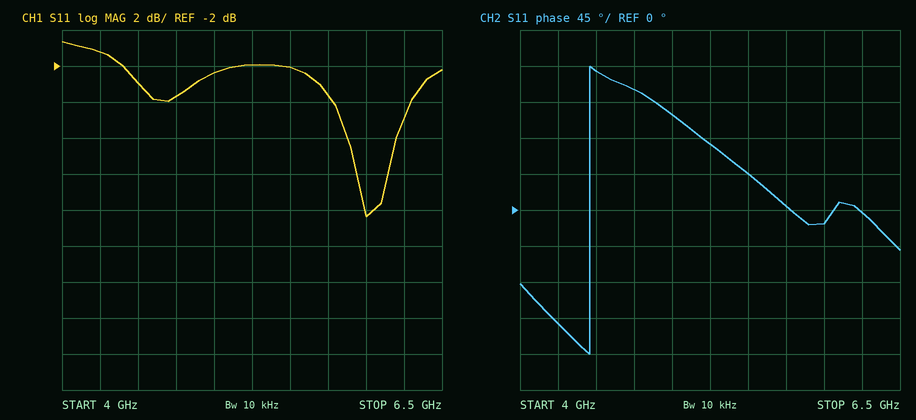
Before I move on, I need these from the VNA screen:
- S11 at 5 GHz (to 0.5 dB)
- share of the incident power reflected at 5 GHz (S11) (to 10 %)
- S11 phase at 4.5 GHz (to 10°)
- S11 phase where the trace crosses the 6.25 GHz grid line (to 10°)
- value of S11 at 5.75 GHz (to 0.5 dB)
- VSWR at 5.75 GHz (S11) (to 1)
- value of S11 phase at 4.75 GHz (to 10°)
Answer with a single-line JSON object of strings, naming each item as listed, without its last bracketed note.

{"S11 at 5 GHz": "-2.5 dB", "share of the incident power reflected at 5 GHz (S11)": "60 %", "S11 phase at 4.5 GHz": "170°", "S11 phase where the trace crosses the 6.25 GHz grid line": "0°", "value of S11 at 5.75 GHz": "-3.5 dB", "VSWR at 5.75 GHz (S11)": "5", "value of S11 phase at 4.75 GHz": "150°"}
